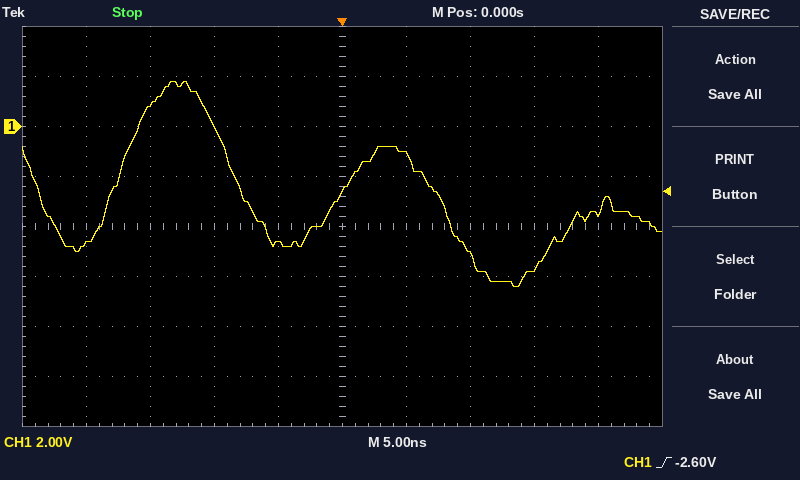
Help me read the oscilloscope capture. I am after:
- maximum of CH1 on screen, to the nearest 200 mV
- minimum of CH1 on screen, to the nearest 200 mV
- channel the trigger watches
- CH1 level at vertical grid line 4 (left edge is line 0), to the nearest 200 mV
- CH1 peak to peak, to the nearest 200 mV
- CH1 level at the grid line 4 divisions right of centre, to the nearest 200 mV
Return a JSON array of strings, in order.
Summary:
["1.8 V", "-6.4 V", "CH1", "-4.6 V", "8.2 V", "-3.4 V"]
